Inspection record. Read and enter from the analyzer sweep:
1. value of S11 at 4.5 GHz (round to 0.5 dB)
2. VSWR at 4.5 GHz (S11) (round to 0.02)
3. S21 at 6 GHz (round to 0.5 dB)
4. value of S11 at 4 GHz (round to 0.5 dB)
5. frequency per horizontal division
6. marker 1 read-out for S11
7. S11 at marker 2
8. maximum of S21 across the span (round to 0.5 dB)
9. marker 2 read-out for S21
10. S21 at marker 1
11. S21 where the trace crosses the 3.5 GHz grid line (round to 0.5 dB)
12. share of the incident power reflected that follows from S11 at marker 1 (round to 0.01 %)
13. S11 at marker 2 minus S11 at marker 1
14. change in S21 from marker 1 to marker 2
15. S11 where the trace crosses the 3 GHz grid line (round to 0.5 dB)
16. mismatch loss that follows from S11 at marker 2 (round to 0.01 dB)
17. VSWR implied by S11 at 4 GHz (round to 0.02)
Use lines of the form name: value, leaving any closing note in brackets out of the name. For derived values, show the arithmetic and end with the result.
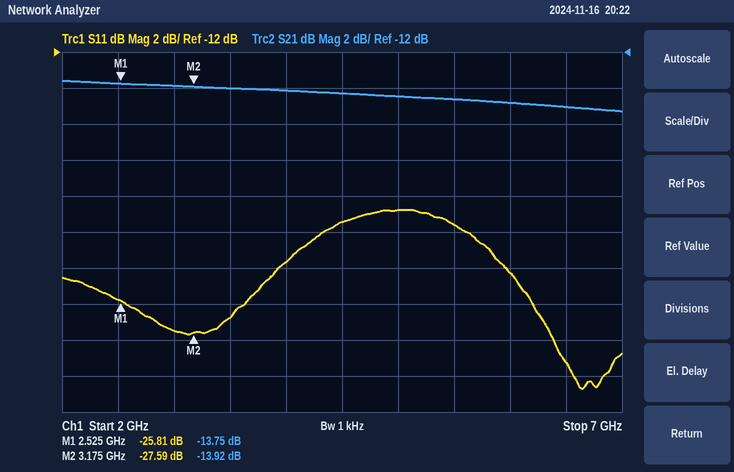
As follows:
value of S11 at 4.5 GHz: -21.5 dB
VSWR at 4.5 GHz (S11): |Γ| = 10^(-21.5/20) = 0.0841; VSWR = (1 + 0.0841)/(1 − 0.0841) ≈ 1.18
S21 at 6 GHz: -15.0 dB
value of S11 at 4 GHz: -23.5 dB
frequency per horizontal division: 500 MHz
marker 1 read-out for S11: -25.81 dB
S11 at marker 2: -27.59 dB
maximum of S21 across the span: -13.5 dB
marker 2 read-out for S21: -13.92 dB
S21 at marker 1: -13.75 dB
S21 where the trace crosses the 3.5 GHz grid line: -14.0 dB
share of the incident power reflected that follows from S11 at marker 1: 10^(-25.81/10) ≈ 0.26 %
S11 at marker 2 minus S11 at marker 1: -27.59 − (-25.81) = -1.78 dB
change in S21 from marker 1 to marker 2: -13.92 − (-13.75) = -0.17 dB
S11 where the trace crosses the 3 GHz grid line: -27.5 dB
mismatch loss that follows from S11 at marker 2: −10 log10(1 − 10^(-27.59/10)) ≈ 0.01 dB
VSWR implied by S11 at 4 GHz: |Γ| = 10^(-23.5/20) = 0.0668; VSWR = (1 + 0.0668)/(1 − 0.0668) ≈ 1.14
